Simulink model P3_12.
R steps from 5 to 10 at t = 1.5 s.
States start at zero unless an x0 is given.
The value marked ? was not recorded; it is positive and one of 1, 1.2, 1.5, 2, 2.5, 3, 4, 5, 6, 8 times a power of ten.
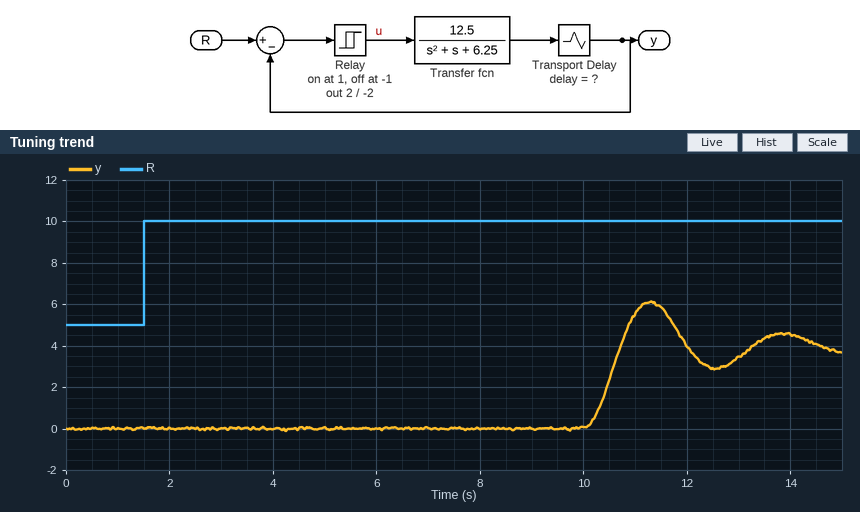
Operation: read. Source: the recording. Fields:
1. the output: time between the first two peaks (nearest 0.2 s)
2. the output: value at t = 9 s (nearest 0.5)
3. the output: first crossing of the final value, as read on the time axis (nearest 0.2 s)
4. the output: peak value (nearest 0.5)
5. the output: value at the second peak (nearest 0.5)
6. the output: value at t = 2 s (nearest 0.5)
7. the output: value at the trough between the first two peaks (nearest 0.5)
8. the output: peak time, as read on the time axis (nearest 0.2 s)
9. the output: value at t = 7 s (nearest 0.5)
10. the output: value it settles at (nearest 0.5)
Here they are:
2.6 s
0.0
10.8 s
6.0
4.5
0.0
3.0
11.2 s
0.0
4.0
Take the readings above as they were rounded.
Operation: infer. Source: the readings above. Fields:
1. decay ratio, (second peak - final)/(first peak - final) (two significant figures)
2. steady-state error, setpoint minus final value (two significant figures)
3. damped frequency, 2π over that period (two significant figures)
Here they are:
0.25
6.0
2.4 rad/s
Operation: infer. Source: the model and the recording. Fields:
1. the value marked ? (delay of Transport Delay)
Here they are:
10
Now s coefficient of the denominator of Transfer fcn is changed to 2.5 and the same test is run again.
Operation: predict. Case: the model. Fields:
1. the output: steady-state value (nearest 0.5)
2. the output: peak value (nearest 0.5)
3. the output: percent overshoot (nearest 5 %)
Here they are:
4.0
4.5
15 %
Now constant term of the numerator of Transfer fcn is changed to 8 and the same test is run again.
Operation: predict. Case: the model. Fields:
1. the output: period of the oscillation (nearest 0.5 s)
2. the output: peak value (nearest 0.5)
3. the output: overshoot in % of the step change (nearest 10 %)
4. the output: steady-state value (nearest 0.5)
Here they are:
2.5 s
4.0
50 %
2.5
